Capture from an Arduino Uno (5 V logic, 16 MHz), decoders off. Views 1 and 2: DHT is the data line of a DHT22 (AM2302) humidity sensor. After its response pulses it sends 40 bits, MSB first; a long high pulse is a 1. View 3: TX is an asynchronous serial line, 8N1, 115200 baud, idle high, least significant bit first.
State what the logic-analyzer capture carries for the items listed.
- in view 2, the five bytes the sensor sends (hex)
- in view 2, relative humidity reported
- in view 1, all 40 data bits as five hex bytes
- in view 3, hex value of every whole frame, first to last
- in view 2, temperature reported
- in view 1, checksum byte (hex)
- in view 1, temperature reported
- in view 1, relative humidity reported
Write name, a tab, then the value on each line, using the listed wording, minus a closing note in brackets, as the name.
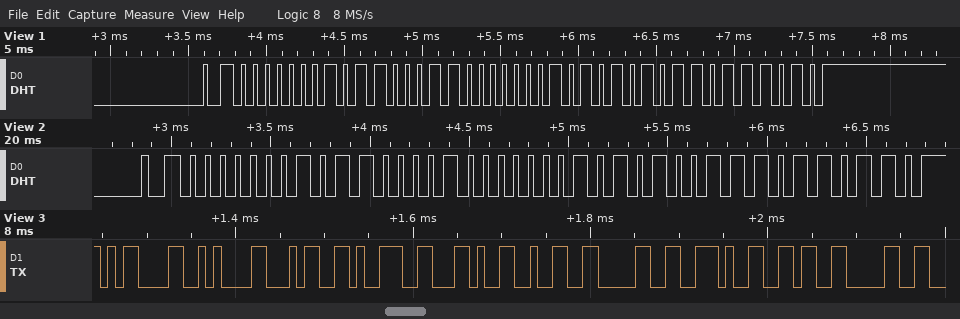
in view 2, the five bytes the sensor sends	01 61 01 53 B6
in view 2, relative humidity reported	35.3 %
in view 1, all 40 data bits as five hex bytes	01 63 01 55 BA
in view 3, hex value of every whole frame, first to last	0x0D 0x0A 0x34 0x39 0x2C 0x32 0x30 0x2E 0x36 0x30
in view 2, temperature reported	33.9 °C
in view 1, checksum byte	0xBA
in view 1, temperature reported	34.1 °C
in view 1, relative humidity reported	35.5 %
